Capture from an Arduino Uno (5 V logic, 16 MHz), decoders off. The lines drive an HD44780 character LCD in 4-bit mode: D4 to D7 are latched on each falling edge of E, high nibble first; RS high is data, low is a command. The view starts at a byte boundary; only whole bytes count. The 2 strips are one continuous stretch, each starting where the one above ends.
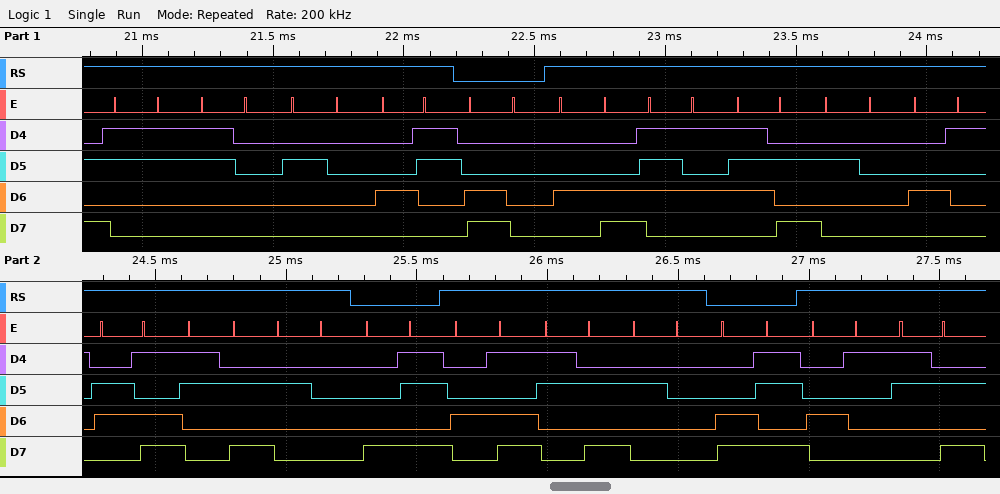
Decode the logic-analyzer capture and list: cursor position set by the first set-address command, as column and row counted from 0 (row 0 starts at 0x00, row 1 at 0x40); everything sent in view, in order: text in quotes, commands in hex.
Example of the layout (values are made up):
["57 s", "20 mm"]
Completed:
["column 0, row 1", "\"30 C\" 0xC0 \"Luz Am: \" 0x8B \"M: \" 0xCB \"A:\""]
